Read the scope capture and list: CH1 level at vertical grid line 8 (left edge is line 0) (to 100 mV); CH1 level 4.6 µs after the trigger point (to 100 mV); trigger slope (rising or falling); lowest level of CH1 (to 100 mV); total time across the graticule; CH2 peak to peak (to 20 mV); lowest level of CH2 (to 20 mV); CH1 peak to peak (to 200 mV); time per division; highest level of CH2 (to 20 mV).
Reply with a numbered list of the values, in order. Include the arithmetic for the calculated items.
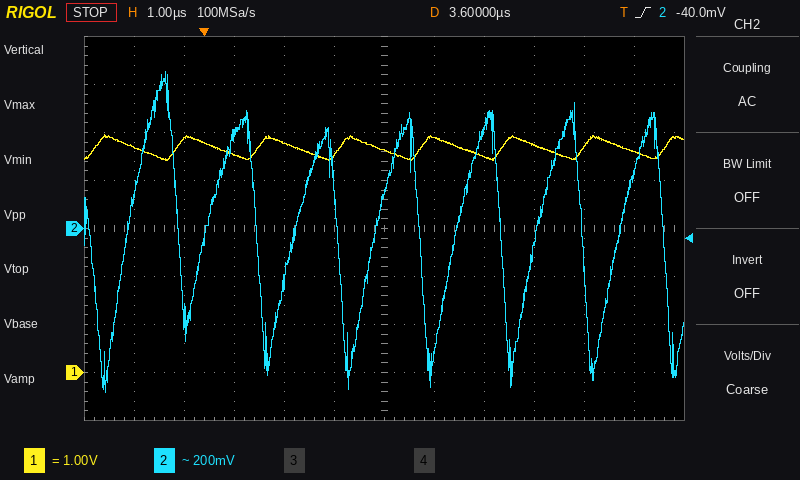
1. 4.5 V
2. 4.9 V
3. rising
4. 4.4 V
5. 12 µs
6. 660 mV − (-680 mV) = 1.34 V
7. -680 mV
8. 600 mV
9. 1 µs
10. 660 mV
